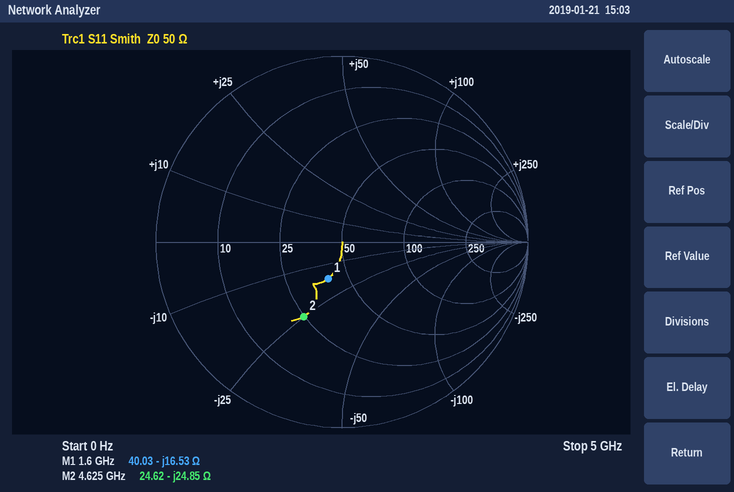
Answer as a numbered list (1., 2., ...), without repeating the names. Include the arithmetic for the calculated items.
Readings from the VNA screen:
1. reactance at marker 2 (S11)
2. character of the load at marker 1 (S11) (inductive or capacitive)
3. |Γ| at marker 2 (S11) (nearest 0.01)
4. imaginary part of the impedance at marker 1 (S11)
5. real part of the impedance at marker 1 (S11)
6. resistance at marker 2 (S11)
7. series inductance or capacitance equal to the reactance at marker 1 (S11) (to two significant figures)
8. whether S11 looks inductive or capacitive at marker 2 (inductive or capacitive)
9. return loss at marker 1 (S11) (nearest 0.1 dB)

1. -24.85 Ω
2. capacitive
3. 0.45
4. -16.53 Ω
5. 40.03 Ω
6. 24.62 Ω
7. C = 1/(2π × 1.6 GHz × 16.53 Ω) ≈ 6.0 pF
8. capacitive
9. 13.5 dB
